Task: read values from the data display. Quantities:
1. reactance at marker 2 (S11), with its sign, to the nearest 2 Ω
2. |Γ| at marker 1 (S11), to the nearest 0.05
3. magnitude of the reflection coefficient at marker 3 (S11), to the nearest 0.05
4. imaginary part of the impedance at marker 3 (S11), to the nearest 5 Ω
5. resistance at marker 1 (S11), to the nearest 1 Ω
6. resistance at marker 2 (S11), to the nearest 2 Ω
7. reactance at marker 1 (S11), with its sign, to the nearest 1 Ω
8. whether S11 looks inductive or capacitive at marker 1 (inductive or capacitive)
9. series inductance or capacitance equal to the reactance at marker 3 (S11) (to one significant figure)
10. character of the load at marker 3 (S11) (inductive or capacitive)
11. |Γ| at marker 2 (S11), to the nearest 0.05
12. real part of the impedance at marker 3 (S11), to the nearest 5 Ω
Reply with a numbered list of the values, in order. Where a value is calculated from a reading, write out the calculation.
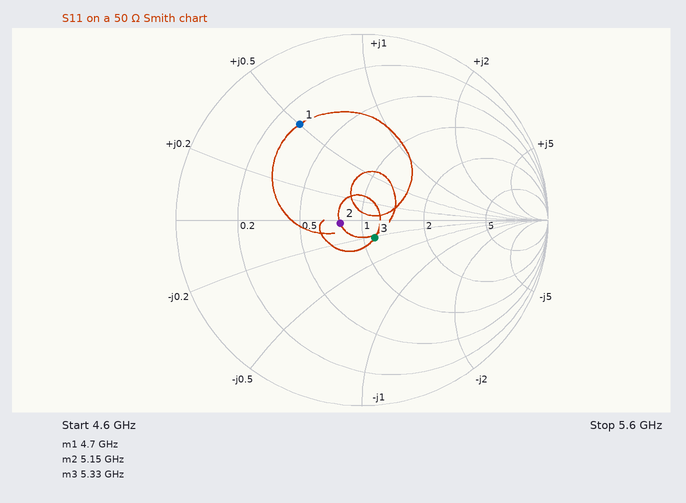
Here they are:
1. -2 Ω
2. 0.60
3. 0.10
4. -10 Ω
5. 15 Ω
6. 40 Ω
7. +25 Ω
8. inductive
9. C = 1/(2π × 5.33 GHz × 10 Ω) ≈ 3 pF
10. capacitive
11. 0.10
12. 55 Ω
